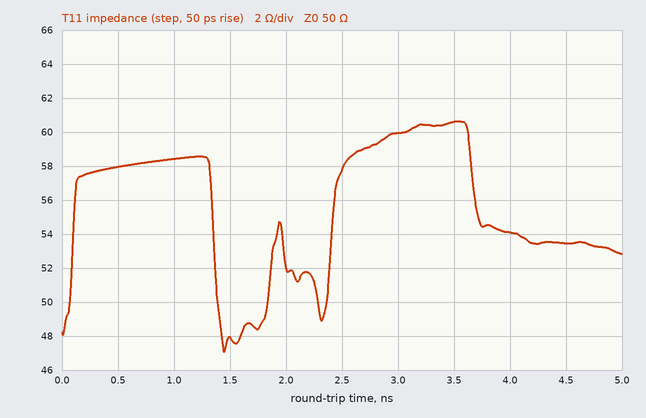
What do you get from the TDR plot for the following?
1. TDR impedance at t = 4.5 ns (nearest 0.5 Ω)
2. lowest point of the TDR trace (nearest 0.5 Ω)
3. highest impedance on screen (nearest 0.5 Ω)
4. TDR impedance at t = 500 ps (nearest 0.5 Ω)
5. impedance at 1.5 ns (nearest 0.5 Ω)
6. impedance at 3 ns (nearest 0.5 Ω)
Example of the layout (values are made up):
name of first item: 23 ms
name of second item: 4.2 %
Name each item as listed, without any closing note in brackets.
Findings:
TDR impedance at t = 4.5 ns: 53.5 Ω
lowest point of the TDR trace: 47.0 Ω
highest impedance on screen: 60.5 Ω
TDR impedance at t = 500 ps: 58.0 Ω
impedance at 1.5 ns: 48.0 Ω
impedance at 3 ns: 60.0 Ω
